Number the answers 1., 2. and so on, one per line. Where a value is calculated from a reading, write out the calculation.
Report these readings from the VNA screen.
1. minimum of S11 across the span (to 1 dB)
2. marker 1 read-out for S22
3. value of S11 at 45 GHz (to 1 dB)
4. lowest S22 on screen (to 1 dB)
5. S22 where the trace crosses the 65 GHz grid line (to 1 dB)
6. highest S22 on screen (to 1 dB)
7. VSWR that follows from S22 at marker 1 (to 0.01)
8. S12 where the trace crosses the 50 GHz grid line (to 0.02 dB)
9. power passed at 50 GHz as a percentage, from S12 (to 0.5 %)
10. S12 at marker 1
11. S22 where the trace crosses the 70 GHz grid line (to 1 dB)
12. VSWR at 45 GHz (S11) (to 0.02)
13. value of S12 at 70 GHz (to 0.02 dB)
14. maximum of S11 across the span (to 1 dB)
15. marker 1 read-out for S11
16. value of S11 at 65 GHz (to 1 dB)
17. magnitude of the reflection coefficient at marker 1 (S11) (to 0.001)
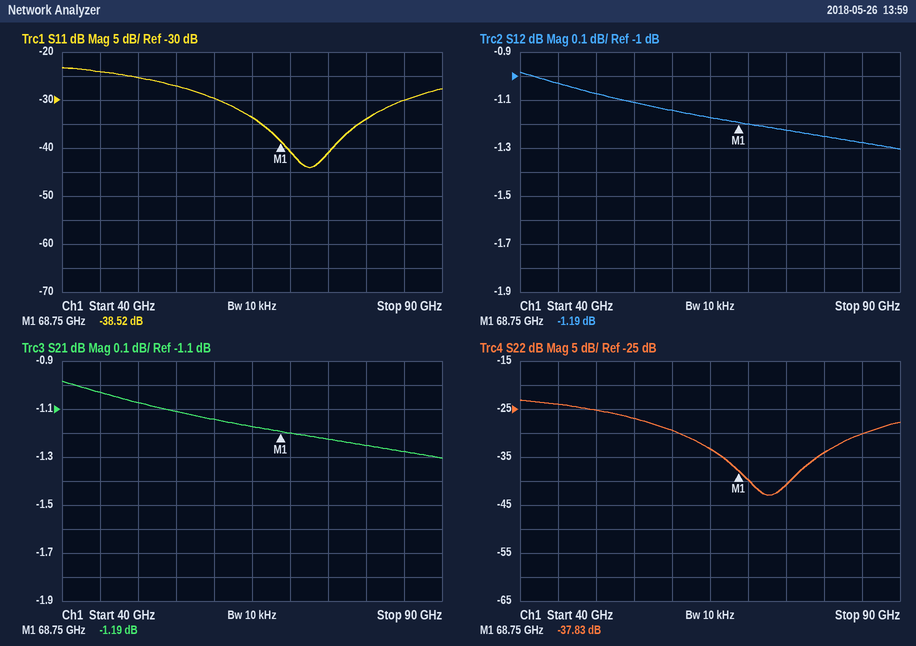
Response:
1. -44 dB
2. -37.83 dB
3. -24 dB
4. -43 dB
5. -33 dB
6. -23 dB
7. (1 + 0.0128)/(1 − 0.0128) ≈ 1.03
8. -1.08 dB
9. 10^(-1.08/10) ≈ 78.0 %
10. -1.19 dB
11. -40 dB
12. |Γ| = 10^(-24/20) = 0.0631; VSWR = (1 + 0.0631)/(1 − 0.0631) ≈ 1.13, so 1.14 to the nearest 0.02
13. -1.20 dB
14. -23 dB
15. -38.52 dB
16. -34 dB
17. 10^(-38.52/20) ≈ 0.012
